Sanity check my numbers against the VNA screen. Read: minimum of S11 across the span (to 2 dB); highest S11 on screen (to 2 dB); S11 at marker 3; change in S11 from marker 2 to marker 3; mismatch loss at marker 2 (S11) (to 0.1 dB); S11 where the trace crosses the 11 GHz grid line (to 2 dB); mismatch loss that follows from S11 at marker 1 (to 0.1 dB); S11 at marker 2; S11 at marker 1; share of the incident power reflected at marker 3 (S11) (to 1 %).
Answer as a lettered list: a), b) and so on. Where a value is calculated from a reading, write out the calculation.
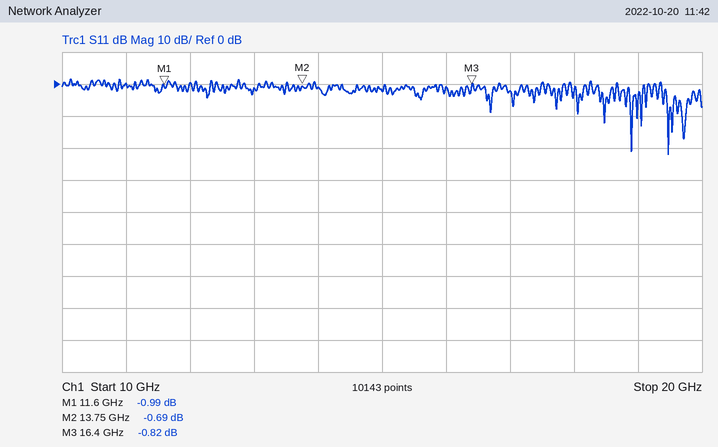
a) -22 dB
b) 2 dB
c) -0.82 dB
d) -0.82 − (-0.69) = -0.13 dB
e) −10 log10(1 − 10^(-0.69/10)) ≈ 8.3 dB
f) 0 dB
g) −10 log10(1 − 10^(-0.99/10)) ≈ 6.9 dB
h) -0.69 dB
i) -0.99 dB
j) 10^(-0.82/10) ≈ 83 %
